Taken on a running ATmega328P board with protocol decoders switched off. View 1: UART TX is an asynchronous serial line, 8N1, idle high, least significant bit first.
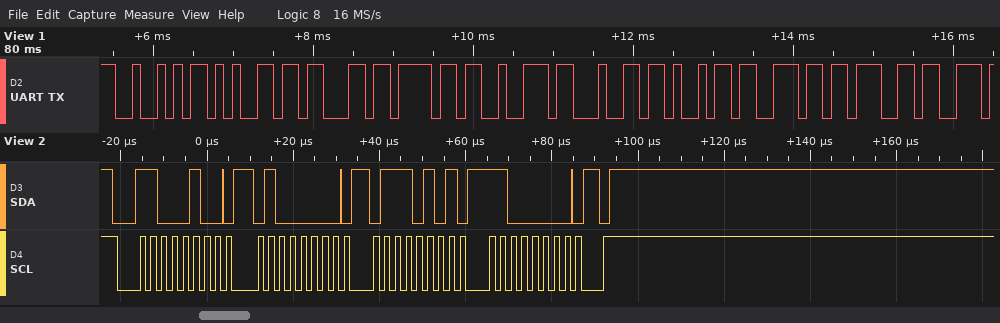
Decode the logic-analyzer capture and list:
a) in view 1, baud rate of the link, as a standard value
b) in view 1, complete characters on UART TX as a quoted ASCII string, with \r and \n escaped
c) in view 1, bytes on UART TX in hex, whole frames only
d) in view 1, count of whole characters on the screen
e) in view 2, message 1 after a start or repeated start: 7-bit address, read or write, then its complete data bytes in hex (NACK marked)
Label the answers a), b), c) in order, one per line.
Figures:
a) 9600 baud
b) "Recording"
c) 52 65 63 6F 72 64 69 6E 67
d) 9
e) 0x62 write: 40 75 C0
